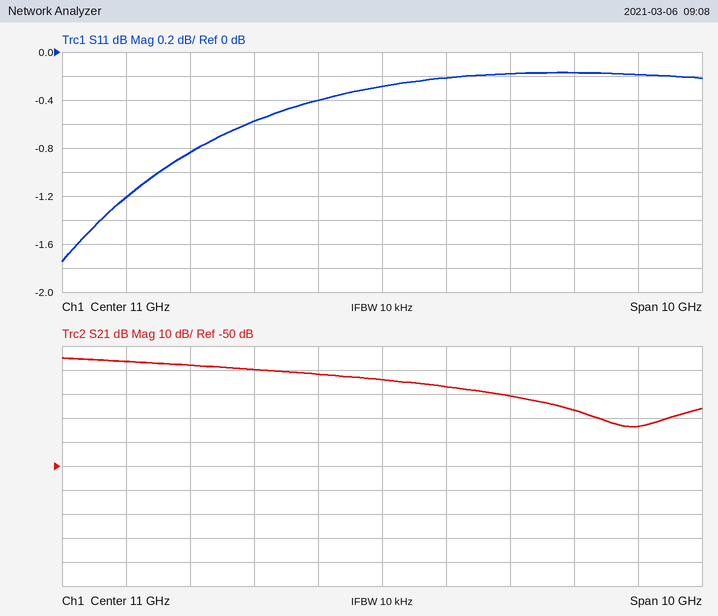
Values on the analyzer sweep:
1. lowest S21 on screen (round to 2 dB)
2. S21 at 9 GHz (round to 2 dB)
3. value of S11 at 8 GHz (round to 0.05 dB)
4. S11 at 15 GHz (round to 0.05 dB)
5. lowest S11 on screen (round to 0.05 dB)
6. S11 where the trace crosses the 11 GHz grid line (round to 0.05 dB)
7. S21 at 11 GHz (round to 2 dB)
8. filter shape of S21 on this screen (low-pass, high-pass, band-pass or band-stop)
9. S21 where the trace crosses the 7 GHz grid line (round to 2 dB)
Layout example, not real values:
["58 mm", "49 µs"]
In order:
["-34 dB", "-10 dB", "-0.85 dB", "-0.20 dB", "-1.75 dB", "-0.30 dB", "-14 dB", "low-pass", "-6 dB"]
